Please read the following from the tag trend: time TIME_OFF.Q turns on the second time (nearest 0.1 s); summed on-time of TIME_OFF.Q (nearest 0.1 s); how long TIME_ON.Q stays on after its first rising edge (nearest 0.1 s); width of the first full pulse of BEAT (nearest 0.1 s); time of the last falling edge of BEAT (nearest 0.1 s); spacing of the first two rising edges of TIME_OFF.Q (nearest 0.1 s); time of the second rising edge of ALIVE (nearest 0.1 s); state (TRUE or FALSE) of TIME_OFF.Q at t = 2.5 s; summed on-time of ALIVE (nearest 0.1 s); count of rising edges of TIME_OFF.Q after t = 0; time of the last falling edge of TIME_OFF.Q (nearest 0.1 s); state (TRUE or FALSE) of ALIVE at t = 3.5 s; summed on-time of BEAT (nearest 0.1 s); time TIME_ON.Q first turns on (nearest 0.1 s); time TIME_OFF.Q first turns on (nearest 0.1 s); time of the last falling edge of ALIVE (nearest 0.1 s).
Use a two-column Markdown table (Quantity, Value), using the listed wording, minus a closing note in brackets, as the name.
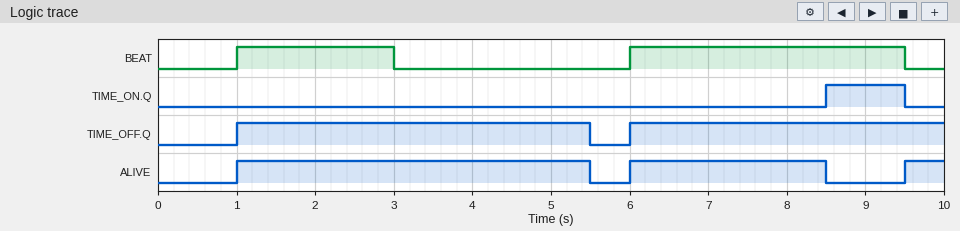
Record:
| Quantity | Value |
|---|---|
| time TIME_OFF.Q turns on the second time | 6.0 s |
| summed on-time of TIME_OFF.Q | 8.5 s |
| how long TIME_ON.Q stays on after its first rising edge | 1.0 s |
| width of the first full pulse of BEAT | 2.0 s |
| time of the last falling edge of BEAT | 9.5 s |
| spacing of the first two rising edges of TIME_OFF.Q | 5.0 s |
| time of the second rising edge of ALIVE | 6.0 s |
| state (TRUE or FALSE) of TIME_OFF.Q at t = 2.5 s | TRUE |
| summed on-time of ALIVE | 7.5 s |
| count of rising edges of TIME_OFF.Q after t = 0 | 2 |
| time of the last falling edge of TIME_OFF.Q | 5.5 s |
| state (TRUE or FALSE) of ALIVE at t = 3.5 s | TRUE |
| summed on-time of BEAT | 5.5 s |
| time TIME_ON.Q first turns on | 8.5 s |
| time TIME_OFF.Q first turns on | 1.0 s |
| time of the last falling edge of ALIVE | 8.5 s |
